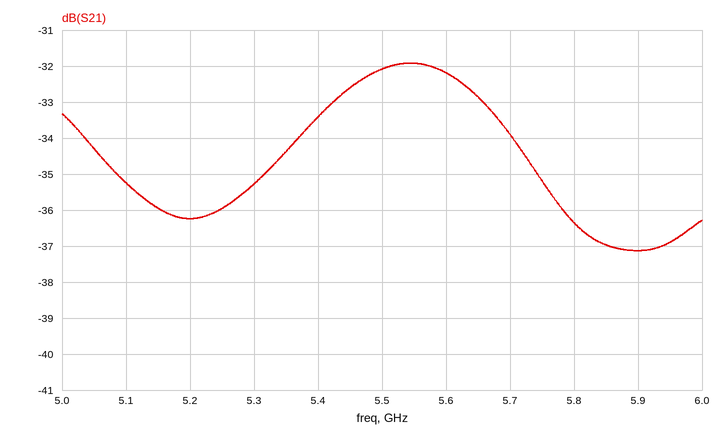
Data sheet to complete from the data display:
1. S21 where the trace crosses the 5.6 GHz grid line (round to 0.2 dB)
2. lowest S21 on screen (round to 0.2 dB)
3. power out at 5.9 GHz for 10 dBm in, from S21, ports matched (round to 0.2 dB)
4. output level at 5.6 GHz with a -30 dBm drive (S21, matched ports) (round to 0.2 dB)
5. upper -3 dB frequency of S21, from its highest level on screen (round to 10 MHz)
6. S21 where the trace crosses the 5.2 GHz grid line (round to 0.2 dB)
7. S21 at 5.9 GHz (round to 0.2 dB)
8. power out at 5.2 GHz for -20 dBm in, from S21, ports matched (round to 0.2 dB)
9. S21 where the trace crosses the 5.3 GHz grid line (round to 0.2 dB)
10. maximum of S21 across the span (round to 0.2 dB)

-32.2 dB
-37.2 dB
-27.2 dBm
-62.2 dBm
5.74 GHz
-36.2 dB
-37.2 dB
-56.2 dBm
-35.2 dB
-32.0 dB
